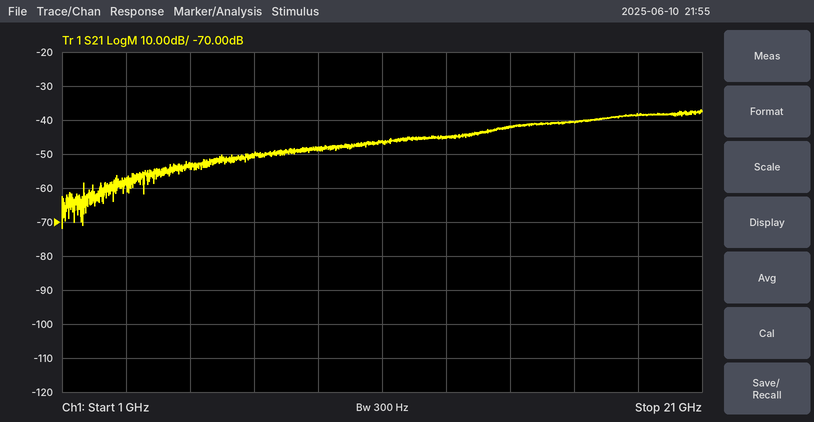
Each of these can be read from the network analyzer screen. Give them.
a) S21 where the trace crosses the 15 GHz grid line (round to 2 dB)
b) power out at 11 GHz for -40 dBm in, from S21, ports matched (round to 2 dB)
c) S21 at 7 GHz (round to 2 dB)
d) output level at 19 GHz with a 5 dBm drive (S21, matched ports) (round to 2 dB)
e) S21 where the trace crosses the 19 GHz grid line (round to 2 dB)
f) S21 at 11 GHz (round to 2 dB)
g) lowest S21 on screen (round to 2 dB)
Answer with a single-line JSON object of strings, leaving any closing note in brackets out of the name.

{"S21 where the trace crosses the 15 GHz grid line": "-42 dB", "power out at 11 GHz for -40 dBm in, from S21, ports matched": "-86 dBm", "S21 at 7 GHz": "-50 dB", "output level at 19 GHz with a 5 dBm drive (S21, matched ports)": "-34 dBm", "S21 where the trace crosses the 19 GHz grid line": "-38 dB", "S21 at 11 GHz": "-46 dB", "lowest S21 on screen": "-72 dB"}
